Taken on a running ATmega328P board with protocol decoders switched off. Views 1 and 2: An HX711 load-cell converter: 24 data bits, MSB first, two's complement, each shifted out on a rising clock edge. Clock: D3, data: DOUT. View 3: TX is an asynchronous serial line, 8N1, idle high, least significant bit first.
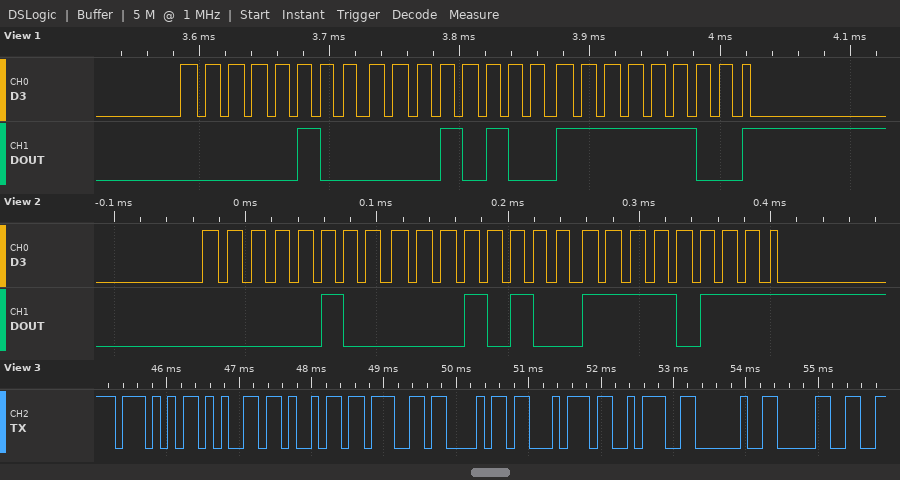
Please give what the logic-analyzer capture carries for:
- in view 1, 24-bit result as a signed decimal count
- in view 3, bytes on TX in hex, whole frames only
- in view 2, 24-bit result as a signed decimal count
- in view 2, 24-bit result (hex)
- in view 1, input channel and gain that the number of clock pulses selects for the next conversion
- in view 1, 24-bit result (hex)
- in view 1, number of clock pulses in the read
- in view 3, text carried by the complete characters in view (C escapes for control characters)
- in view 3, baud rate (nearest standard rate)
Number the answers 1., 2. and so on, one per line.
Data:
1. 267516
2. 57 65 69 67 68 74 3A 20 30
3. 267511
4. 0x0414F7
5. channel A, gain 128
6. 0x0414FC
7. 25
8. "Weight: 0"
9. 9600 baud
